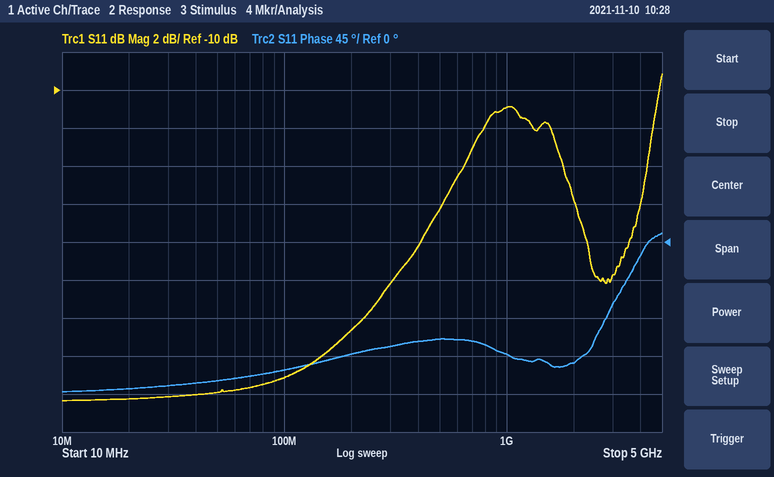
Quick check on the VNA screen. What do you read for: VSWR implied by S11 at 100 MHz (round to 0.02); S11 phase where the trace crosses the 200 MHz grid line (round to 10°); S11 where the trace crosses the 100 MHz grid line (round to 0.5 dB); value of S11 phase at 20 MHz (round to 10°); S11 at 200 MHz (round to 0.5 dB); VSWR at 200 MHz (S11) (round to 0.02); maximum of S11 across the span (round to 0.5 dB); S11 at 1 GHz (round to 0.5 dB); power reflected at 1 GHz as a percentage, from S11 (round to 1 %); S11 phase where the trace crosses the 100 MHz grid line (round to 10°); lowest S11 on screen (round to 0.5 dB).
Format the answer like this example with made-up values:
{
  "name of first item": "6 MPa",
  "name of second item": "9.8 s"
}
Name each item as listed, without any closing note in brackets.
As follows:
{
  "VSWR implied by S11 at 100 MHz": "1.12",
  "S11 phase where the trace crosses the 200 MHz grid line": "-130°",
  "S11 where the trace crosses the 100 MHz grid line": "-25.0 dB",
  "value of S11 phase at 20 MHz": "-170°",
  "S11 at 200 MHz": "-22.5 dB",
  "VSWR at 200 MHz (S11)": "1.16",
  "maximum of S11 across the span": "-9.0 dB",
  "S11 at 1 GHz": "-11.0 dB",
  "power reflected at 1 GHz as a percentage, from S11": "8 %",
  "S11 phase where the trace crosses the 100 MHz grid line": "-150°",
  "lowest S11 on screen": "-26.5 dB"
}
